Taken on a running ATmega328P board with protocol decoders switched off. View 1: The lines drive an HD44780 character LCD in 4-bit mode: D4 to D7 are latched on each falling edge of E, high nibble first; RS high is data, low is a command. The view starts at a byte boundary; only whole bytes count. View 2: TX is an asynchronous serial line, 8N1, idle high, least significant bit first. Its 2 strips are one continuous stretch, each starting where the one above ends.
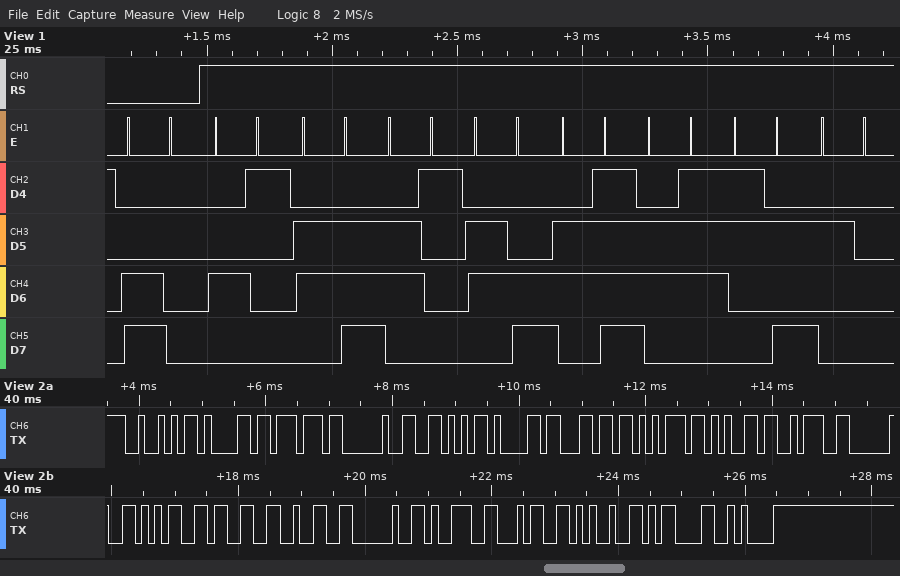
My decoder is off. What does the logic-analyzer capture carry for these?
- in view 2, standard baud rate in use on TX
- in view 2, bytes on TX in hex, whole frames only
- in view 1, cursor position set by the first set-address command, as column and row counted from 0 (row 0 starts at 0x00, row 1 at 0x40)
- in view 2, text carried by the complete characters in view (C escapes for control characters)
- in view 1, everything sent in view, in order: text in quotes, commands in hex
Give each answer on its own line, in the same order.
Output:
9600 baud
52 61 77 20 56 61 6C 75 65 3A 20 35 33 32 20 39 34 25 0D 0A
column 0, row 1
"Raw Value: 532 94%\r\n"
0xC0 "Analog: "
